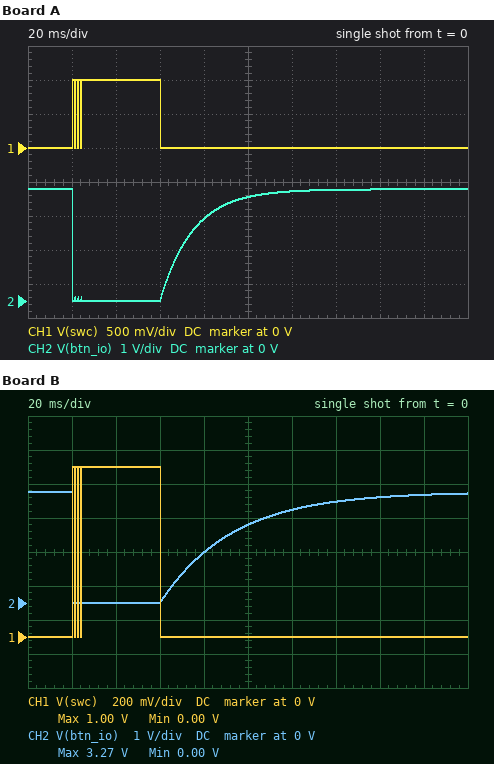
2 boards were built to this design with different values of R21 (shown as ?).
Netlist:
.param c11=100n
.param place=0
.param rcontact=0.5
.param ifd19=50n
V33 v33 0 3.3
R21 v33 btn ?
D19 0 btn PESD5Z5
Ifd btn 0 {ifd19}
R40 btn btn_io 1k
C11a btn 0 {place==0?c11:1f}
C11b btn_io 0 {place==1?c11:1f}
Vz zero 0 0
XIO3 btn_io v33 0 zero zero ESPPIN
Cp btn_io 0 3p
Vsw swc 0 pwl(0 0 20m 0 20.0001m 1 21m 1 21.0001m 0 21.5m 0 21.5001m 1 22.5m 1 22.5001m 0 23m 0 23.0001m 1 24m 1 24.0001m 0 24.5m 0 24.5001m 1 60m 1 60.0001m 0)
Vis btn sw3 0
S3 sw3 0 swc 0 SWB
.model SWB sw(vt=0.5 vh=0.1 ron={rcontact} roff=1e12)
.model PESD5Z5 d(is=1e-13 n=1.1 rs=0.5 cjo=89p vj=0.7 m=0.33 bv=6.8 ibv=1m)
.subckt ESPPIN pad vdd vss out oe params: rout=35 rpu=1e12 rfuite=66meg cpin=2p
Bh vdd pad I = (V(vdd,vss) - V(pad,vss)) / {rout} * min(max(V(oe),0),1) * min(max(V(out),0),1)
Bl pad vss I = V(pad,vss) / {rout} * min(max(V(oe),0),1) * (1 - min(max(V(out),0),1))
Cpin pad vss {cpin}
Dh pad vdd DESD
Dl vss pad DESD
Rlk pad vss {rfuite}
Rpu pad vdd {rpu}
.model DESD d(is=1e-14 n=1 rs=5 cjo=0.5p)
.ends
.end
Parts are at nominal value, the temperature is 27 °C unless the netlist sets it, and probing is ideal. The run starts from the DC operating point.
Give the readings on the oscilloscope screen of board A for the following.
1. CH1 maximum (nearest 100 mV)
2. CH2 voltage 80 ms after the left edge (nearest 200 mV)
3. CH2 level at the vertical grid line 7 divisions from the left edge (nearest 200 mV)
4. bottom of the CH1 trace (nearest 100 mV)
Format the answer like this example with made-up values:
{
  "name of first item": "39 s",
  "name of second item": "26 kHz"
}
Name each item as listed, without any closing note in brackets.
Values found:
{
  "CH1 maximum": "1.0 V",
  "CH2 voltage 80 ms after the left edge": "2.4 V",
  "CH2 level at the vertical grid line 7 divisions from the left edge": "3.2 V",
  "bottom of the CH1 trace": "0 V"
}
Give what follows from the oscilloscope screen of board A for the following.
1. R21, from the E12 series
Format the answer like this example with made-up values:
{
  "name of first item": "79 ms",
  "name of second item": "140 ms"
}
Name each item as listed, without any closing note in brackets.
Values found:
{
  "R21, from the E12 series": "150 kΩ"
}
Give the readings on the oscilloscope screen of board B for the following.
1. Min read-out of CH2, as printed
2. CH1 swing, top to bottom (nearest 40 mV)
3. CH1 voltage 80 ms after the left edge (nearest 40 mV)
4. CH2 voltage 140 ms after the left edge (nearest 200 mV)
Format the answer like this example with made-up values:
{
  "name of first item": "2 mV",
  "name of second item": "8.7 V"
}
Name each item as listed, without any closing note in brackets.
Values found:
{
  "Min read-out of CH2, as printed": "0.00 V",
  "CH1 swing, top to bottom": "1.00 V",
  "CH1 voltage 80 ms after the left edge": "0 V",
  "CH2 voltage 140 ms after the left edge": "3.0 V"
}
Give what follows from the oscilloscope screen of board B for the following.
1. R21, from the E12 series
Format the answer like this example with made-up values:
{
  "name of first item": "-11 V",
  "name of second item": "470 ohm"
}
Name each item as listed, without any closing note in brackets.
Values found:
{
  "R21, from the E12 series": "330 kΩ"
}
